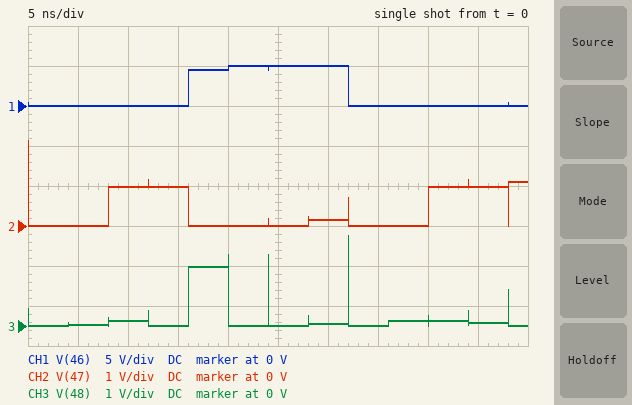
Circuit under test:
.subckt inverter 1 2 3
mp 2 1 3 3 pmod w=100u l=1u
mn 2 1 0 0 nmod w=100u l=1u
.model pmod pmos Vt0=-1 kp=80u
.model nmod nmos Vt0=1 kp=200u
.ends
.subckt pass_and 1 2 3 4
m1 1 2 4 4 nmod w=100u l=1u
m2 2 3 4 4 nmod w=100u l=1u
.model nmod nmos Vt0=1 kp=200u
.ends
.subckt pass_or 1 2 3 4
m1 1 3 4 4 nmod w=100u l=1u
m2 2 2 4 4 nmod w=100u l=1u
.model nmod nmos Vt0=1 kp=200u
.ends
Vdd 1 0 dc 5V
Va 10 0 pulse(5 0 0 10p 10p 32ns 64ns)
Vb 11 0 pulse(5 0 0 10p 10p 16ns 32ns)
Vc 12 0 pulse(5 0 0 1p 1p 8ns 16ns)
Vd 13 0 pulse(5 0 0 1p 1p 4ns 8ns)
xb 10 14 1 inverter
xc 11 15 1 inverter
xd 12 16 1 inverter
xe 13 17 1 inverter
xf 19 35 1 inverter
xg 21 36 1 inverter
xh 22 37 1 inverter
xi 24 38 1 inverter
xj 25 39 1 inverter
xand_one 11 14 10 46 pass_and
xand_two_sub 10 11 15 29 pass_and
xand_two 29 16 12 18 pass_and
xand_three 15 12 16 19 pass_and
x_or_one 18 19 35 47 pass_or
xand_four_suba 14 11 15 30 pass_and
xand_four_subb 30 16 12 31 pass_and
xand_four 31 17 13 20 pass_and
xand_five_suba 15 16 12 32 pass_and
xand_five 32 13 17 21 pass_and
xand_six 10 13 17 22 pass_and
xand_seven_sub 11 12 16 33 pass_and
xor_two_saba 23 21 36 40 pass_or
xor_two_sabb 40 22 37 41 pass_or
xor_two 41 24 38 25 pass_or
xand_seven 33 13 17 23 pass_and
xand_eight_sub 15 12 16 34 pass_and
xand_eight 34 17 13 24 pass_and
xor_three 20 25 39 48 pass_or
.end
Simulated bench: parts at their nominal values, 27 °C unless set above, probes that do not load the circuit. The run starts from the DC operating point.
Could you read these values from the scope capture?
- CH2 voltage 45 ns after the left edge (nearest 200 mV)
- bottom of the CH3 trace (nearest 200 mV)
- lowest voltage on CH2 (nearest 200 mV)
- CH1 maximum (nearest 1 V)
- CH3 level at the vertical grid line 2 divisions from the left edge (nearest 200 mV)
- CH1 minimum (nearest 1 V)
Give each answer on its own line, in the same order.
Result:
1.0 V
0 V
0 V
5 V
200 mV
0 V
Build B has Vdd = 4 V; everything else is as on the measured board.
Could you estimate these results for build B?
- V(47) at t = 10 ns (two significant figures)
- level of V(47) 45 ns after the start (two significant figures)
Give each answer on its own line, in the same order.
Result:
940 mV
960 mV
